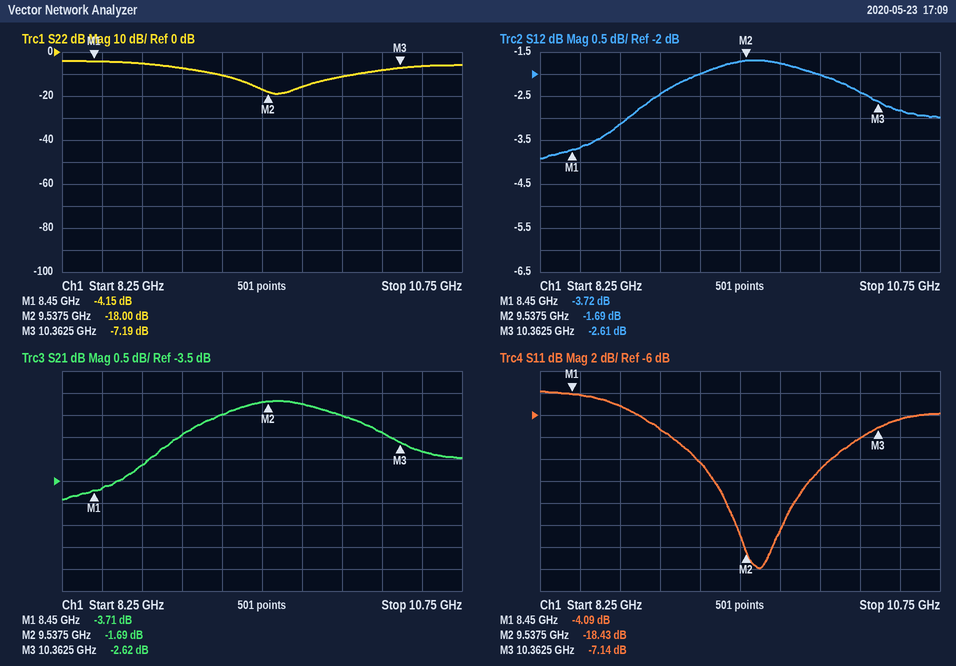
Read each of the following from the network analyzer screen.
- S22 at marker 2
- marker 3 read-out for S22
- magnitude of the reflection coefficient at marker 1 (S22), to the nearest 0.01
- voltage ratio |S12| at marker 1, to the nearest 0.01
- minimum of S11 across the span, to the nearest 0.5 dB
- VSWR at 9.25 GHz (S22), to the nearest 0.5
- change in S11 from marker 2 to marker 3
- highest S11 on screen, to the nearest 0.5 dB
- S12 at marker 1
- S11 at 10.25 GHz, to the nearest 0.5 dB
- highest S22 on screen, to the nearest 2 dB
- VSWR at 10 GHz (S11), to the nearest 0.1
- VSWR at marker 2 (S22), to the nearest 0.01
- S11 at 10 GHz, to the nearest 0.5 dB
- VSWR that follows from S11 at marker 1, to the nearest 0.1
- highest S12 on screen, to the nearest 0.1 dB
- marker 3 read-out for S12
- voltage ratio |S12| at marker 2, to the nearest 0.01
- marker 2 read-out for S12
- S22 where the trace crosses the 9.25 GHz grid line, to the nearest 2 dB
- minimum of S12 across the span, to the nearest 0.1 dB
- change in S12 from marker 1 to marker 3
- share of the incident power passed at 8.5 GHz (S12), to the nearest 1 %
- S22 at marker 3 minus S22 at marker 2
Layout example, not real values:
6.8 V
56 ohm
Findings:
-18.00 dB
-7.19 dB
0.62
0.65
-20.0 dB
2.0
11.29 dB
-4.0 dB
-3.72 dB
-8.0 dB
-4 dB
1.8
1.29
-11.0 dB
4.3
-1.7 dB
-2.61 dB
0.82
-1.69 dB
-10 dB
-3.9 dB
1.11 dB
43 %
10.81 dB
